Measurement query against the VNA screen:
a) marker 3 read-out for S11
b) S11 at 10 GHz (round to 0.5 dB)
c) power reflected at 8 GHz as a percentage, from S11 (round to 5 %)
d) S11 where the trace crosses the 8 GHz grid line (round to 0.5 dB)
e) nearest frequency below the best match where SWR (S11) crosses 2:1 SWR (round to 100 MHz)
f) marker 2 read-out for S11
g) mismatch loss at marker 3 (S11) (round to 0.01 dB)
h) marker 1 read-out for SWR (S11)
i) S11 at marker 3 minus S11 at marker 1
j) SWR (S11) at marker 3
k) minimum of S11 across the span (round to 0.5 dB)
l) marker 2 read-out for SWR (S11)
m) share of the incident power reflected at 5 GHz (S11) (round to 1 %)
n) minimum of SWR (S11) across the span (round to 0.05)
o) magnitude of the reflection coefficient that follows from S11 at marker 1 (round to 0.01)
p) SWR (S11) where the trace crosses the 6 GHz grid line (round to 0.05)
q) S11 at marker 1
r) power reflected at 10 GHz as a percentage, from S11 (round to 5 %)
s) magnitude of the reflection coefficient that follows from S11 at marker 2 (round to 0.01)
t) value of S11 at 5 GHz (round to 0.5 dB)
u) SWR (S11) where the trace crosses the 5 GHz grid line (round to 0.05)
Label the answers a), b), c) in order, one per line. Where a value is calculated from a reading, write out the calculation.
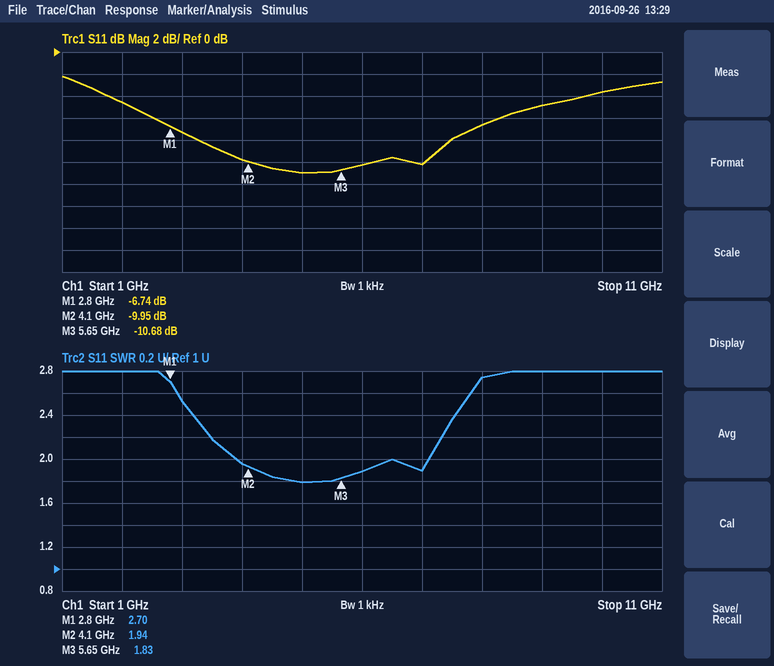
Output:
a) -10.68 dB
b) -3.5 dB
c) 10^(-6.5/10) ≈ 22.4 %, so 20 % to the nearest 5 %
d) -6.5 dB
e) 3.9 GHz
f) -9.95 dB
g) −10 log10(1 − 10^(-10.68/10)) ≈ 0.39 dB
h) 2.70
i) -10.68 − (-6.74) = -3.94 dB
j) 1.83
k) -11.0 dB
l) 1.94
m) 10^(-11/10) ≈ 8 %
n) 1.80
o) 10^(-6.74/20) ≈ 0.46
p) 1.90
q) -6.74 dB
r) 10^(-3.5/10) ≈ 45 %
s) 10^(-9.95/20) ≈ 0.32
t) -11.0 dB
u) 1.80
